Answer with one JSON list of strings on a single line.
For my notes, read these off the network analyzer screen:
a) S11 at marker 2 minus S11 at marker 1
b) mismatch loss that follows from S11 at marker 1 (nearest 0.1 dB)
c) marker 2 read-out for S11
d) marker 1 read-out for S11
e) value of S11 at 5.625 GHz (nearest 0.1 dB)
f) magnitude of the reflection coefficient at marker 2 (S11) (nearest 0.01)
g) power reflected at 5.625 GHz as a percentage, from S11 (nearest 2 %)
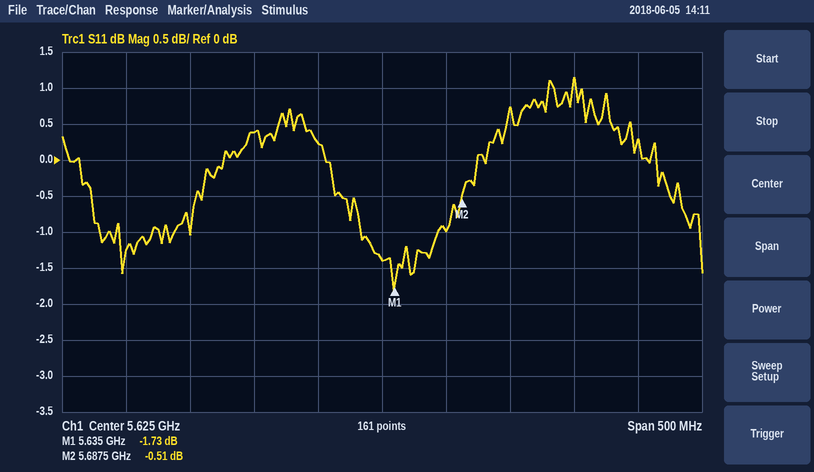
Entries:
["1.22 dB", "4.8 dB", "-0.51 dB", "-1.73 dB", "-1.4 dB", "0.94", "72 %"]
